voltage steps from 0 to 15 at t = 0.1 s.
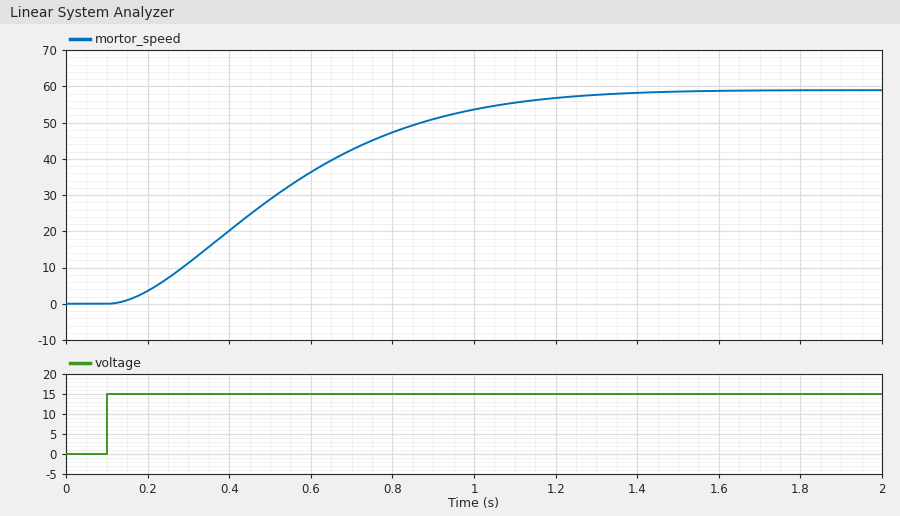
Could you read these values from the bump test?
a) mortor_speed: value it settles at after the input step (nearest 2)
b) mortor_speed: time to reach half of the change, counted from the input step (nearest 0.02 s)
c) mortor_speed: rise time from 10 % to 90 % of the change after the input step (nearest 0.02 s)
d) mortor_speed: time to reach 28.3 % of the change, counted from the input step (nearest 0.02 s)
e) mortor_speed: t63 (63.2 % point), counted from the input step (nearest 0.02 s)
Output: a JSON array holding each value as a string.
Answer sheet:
["58", "0.40 s", "0.74 s", "0.26 s", "0.52 s"]
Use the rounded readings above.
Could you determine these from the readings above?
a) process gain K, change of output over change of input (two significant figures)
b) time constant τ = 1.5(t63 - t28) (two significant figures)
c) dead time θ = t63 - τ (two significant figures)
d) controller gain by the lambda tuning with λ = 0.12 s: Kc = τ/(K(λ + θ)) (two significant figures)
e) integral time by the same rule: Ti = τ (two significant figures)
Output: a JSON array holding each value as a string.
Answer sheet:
["3.9", "0.39 s", "0.13 s", "0.40", "0.39 s"]
